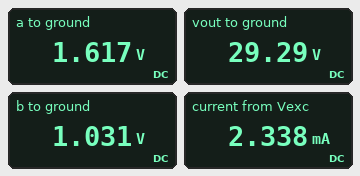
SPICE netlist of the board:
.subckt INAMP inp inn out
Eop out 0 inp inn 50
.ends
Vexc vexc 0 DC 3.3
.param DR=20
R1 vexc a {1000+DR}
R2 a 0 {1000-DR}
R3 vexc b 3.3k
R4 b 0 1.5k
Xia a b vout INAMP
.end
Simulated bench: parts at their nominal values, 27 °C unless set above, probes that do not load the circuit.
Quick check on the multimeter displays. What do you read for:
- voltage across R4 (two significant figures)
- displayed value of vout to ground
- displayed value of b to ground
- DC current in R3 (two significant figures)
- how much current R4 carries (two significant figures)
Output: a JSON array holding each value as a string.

["1.0 V", "29.29 V", "1.031 V", "690 µA", "690 µA"]
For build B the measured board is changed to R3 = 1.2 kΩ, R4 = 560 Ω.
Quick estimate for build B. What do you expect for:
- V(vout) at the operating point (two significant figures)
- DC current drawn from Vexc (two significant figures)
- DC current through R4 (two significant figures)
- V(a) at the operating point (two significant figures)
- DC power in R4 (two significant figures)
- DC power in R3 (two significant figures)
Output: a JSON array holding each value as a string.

["28 V", "3.5 mA", "1.9 mA", "1.6 V", "2.0 mW", "4.2 mW"]
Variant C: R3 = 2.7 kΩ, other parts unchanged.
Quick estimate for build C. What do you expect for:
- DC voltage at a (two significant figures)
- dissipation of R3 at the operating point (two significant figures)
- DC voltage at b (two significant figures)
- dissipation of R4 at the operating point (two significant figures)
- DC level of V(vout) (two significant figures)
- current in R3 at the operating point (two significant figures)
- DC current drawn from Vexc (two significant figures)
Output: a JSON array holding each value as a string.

["1.6 V", "1.7 mW", "1.2 V", "930 µW", "22 V", "790 µA", "2.4 mA"]
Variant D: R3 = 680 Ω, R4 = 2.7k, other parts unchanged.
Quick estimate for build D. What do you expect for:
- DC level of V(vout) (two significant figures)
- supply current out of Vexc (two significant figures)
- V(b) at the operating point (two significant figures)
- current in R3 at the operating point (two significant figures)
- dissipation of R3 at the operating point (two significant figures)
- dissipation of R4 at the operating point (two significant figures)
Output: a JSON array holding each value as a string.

["-51 V", "2.6 mA", "2.6 V", "980 µA", "650 µW", "2.6 mW"]
